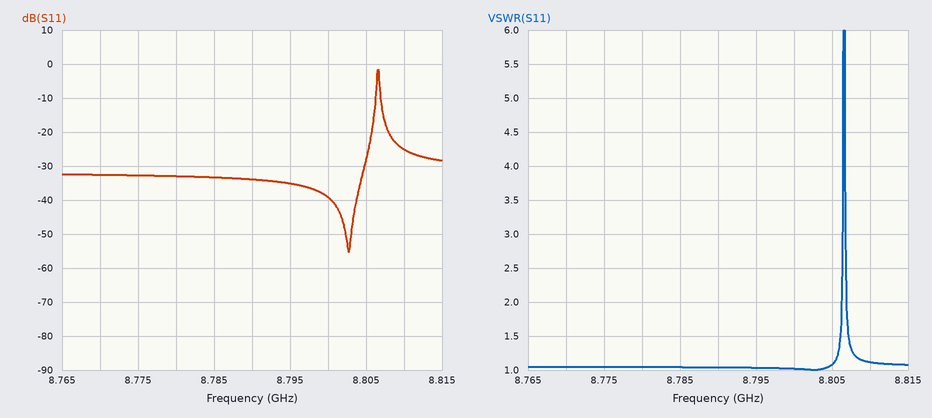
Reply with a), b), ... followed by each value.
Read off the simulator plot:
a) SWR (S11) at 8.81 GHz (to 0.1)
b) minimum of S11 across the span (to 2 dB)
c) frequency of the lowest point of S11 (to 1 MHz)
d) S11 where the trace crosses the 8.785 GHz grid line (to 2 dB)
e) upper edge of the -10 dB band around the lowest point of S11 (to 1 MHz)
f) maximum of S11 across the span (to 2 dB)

a) 1.1
b) -56 dB
c) 8.803 GHz
d) -34 dB
e) 8.806 GHz
f) -2 dB
